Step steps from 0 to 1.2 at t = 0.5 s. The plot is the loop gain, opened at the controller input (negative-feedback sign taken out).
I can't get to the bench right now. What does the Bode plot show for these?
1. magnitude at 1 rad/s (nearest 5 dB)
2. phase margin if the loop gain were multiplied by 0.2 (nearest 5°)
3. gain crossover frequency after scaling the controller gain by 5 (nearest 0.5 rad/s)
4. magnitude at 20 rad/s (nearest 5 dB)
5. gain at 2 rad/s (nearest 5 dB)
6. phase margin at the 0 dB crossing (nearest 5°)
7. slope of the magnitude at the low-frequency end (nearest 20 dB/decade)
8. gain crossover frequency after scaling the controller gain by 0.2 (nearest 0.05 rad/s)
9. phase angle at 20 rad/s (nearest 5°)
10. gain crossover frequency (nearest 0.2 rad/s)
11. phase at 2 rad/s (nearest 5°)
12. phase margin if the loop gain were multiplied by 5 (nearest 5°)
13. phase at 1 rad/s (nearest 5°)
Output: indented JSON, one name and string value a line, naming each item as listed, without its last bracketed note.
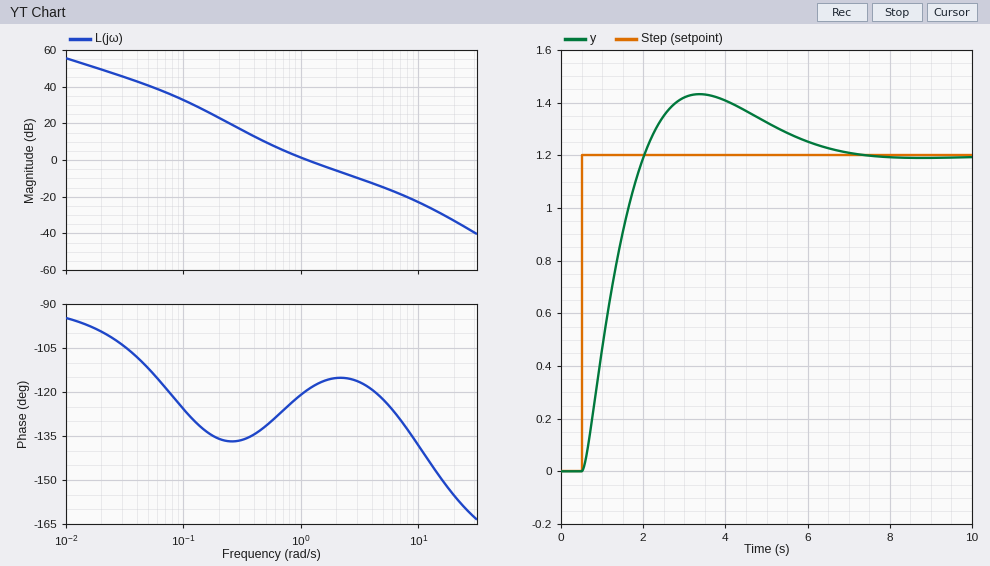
{
  "magnitude at 1 rad/s": "0 dB",
  "phase margin if the loop gain were multiplied by 0.2": "45°",
  "gain crossover frequency after scaling the controller gain by 5": "4.5 rad/s",
  "magnitude at 20 rad/s": "-35 dB",
  "gain at 2 rad/s": "-5 dB",
  "phase margin at the 0 dB crossing": "60°",
  "slope of the magnitude at the low-frequency end": "-20 dB/decade",
  "gain crossover frequency after scaling the controller gain by 0.2": "0.35 rad/s",
  "phase angle at 20 rad/s": "-155°",
  "gain crossover frequency": "1.2 rad/s",
  "phase at 2 rad/s": "-115°",
  "phase margin if the loop gain were multiplied by 5": "60°",
  "phase at 1 rad/s": "-120°"
}
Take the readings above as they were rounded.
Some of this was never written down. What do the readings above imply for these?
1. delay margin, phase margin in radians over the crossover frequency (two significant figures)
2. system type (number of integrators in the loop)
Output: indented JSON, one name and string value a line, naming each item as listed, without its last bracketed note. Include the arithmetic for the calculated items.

{
  "delay margin, phase margin in radians over the crossover frequency": "60 × π / 180 / 1.2 = 0.87 s",
  "system type": "1"
}
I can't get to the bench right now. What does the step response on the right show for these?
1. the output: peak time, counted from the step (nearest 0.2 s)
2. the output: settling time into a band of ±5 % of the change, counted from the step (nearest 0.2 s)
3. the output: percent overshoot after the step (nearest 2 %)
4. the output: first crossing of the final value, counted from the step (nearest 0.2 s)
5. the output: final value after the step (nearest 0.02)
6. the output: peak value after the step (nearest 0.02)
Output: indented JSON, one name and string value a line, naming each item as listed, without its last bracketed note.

{
  "the output: peak time, counted from the step": "2.8 s",
  "the output: settling time into a band of ±5 % of the change, counted from the step": "5.4 s",
  "the output: percent overshoot after the step": "20 %",
  "the output: first crossing of the final value, counted from the step": "1.6 s",
  "the output: final value after the step": "1.20",
  "the output: peak value after the step": "1.44"
}
